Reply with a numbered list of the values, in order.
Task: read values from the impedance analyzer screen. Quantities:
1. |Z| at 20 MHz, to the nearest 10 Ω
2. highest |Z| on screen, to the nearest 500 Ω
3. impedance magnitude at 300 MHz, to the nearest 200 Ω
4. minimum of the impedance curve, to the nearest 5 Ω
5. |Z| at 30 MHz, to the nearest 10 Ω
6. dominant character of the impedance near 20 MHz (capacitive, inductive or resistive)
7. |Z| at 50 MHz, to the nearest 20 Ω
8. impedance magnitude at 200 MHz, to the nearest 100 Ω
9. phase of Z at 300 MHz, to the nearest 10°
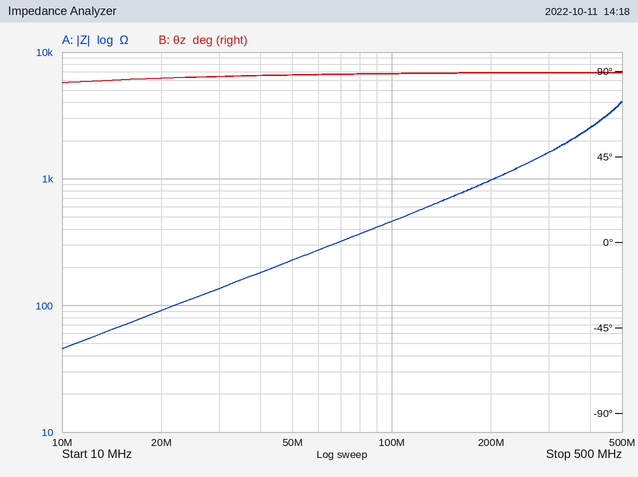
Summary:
1. 90 Ω
2. 4.0 kΩ
3. 1.6 kΩ
4. 45 Ω
5. 140 Ω
6. inductive
7. 220 Ω
8. 1.0 kΩ
9. 90°
